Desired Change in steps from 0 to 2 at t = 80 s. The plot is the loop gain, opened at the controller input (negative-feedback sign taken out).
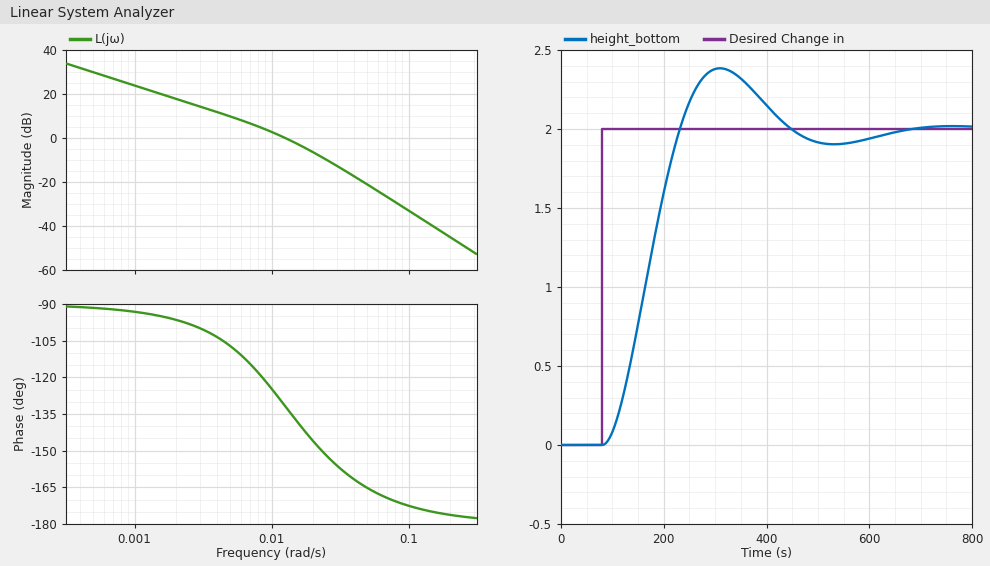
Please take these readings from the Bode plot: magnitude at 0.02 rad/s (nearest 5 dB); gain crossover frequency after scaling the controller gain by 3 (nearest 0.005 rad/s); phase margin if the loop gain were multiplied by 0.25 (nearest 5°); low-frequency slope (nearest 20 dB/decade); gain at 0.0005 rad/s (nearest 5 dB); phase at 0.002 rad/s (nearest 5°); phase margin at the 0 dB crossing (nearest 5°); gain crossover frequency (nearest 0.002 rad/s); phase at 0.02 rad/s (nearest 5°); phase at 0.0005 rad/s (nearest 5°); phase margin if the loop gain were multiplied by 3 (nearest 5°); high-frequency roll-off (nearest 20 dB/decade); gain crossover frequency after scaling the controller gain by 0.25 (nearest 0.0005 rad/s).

-5 dB
0.025 rad/s
75°
-20 dB/decade
30 dB
-95°
50°
0.012 rad/s
-145°
-90°
30°
-40 dB/decade
0.0040 rad/s
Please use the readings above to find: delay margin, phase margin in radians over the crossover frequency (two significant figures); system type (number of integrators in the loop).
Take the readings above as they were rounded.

73 s
1
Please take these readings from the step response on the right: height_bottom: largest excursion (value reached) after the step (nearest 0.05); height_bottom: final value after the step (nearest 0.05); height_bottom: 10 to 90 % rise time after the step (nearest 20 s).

2.40
2.00
100 s
